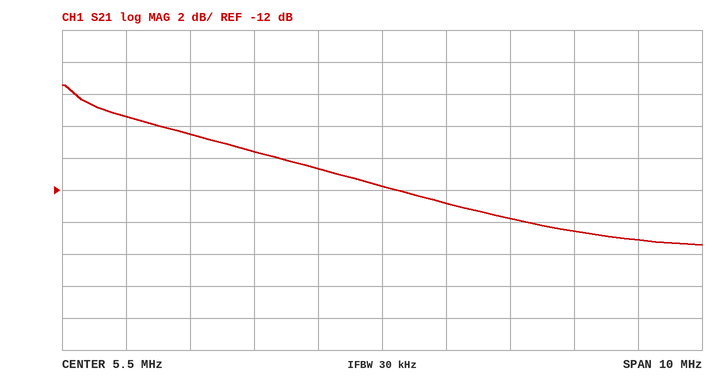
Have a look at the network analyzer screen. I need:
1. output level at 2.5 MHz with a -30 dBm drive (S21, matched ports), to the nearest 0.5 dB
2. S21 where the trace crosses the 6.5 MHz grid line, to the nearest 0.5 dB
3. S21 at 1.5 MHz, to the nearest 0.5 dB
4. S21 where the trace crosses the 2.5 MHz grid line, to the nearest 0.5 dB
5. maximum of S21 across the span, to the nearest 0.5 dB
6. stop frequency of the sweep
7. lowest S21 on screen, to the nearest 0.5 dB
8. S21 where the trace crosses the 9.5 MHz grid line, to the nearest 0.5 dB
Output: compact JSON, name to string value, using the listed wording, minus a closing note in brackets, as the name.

{"output level at 2.5 MHz with a -30 dBm drive (S21, matched ports), to the nearest 0.5 dB": "-38.5 dBm", "S21 where the trace crosses the 6.5 MHz grid line, to the nearest 0.5 dB": "-13.0 dB", "S21 at 1.5 MHz, to the nearest 0.5 dB": "-7.5 dB", "S21 where the trace crosses the 2.5 MHz grid line, to the nearest 0.5 dB": "-8.5 dB", "maximum of S21 across the span, to the nearest 0.5 dB": "-5.5 dB", "stop frequency of the sweep": "10.5 MHz", "lowest S21 on screen, to the nearest 0.5 dB": "-15.5 dB", "S21 where the trace crosses the 9.5 MHz grid line, to the nearest 0.5 dB": "-15.0 dB"}
